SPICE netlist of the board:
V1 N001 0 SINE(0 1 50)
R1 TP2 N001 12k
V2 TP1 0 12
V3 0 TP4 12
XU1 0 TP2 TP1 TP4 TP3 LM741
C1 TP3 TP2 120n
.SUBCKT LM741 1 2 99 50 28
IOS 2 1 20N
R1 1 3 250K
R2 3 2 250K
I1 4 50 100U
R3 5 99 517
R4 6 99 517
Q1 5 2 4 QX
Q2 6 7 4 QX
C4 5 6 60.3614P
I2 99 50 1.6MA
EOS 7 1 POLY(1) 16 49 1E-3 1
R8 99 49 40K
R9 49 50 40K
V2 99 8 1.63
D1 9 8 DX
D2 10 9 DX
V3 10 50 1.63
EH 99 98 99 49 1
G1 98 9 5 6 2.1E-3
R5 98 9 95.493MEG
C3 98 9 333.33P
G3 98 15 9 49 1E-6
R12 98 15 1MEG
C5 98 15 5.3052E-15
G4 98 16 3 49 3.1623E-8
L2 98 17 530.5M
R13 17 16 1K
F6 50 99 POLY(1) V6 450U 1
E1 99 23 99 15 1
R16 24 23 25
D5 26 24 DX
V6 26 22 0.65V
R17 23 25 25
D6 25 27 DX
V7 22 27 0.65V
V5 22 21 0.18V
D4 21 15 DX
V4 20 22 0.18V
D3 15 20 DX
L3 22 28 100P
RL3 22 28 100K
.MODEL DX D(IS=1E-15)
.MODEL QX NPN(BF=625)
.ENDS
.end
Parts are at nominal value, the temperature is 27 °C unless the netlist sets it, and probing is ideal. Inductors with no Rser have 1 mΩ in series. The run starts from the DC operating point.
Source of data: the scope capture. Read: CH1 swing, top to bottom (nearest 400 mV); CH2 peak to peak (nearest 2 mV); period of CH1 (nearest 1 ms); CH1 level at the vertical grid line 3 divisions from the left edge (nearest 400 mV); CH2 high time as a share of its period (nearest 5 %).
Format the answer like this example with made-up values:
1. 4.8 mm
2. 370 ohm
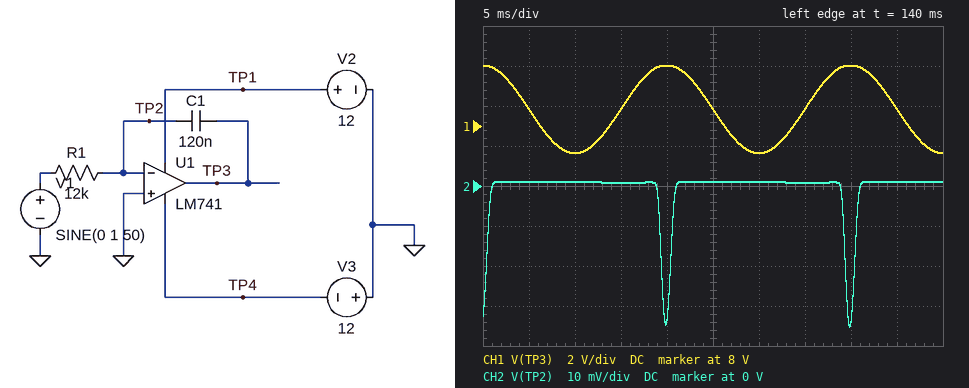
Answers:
1. 4.4 V
2. 36 mV
3. 20 ms
4. 8.8 V
5. 95 %
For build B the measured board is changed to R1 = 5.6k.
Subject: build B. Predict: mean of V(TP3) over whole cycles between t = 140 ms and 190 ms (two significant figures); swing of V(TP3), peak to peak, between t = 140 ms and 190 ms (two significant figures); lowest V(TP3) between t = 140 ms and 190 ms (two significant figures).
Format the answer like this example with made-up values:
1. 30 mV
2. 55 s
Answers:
1. 6.3 V
2. 9.4 V
3. 1.6 V
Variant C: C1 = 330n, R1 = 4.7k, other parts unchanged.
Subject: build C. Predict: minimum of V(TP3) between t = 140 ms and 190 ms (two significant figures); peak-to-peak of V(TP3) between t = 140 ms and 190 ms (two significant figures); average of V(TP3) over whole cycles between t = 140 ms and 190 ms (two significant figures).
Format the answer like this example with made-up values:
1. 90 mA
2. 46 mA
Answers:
1. 6.9 V
2. 4.1 V
3. 9.0 V
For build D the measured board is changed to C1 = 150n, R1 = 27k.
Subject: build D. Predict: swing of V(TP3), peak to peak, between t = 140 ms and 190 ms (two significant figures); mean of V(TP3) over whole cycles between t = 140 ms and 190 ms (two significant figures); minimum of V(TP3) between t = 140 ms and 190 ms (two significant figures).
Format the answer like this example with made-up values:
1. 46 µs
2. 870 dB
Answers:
1. 1.5 V
2. 10 V
3. 9.5 V
